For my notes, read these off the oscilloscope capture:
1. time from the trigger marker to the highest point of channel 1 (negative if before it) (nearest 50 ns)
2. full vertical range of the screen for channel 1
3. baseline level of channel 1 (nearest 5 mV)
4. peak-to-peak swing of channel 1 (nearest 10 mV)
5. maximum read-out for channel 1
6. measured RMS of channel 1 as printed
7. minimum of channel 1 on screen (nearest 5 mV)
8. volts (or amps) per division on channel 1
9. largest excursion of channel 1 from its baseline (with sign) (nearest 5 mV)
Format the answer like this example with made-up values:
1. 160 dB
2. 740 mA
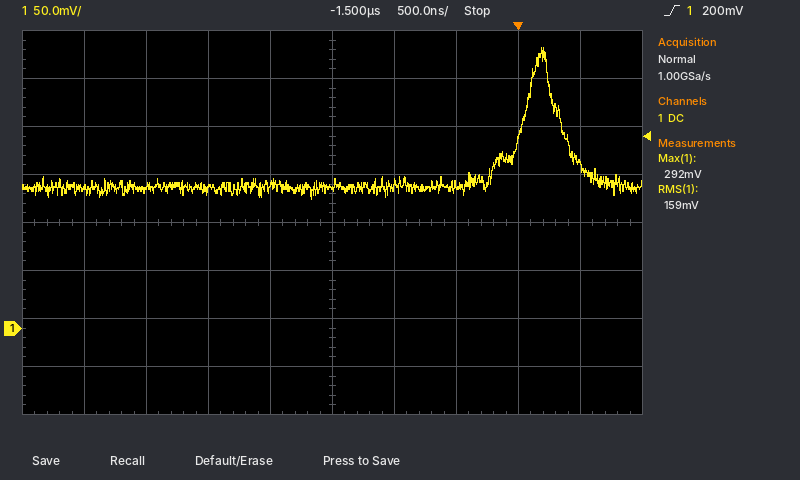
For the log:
1. +200 ns
2. 400 mV
3. 145 mV
4. 160 mV
5. 292 mV
6. 159 mV
7. 135 mV
8. 50 mV
9. +145 mV
